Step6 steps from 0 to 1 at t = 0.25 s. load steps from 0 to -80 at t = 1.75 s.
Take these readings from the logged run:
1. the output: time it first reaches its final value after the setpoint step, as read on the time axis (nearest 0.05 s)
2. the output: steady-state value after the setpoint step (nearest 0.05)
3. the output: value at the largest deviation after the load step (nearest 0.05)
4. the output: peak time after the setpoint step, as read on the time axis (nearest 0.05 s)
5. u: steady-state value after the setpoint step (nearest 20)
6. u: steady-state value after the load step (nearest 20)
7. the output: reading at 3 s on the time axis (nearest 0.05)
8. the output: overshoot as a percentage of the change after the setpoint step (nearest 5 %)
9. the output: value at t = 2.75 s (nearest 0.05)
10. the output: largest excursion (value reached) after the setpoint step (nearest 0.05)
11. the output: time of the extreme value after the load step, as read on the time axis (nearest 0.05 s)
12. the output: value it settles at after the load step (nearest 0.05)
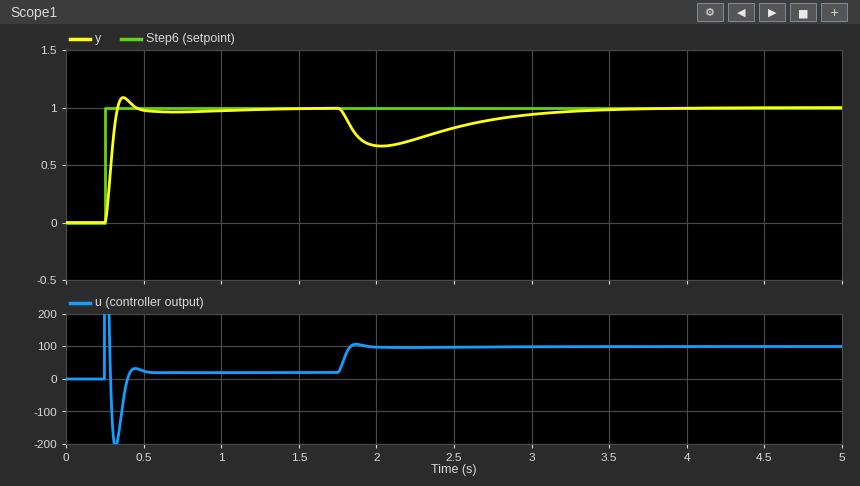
0.35 s
1.00
0.65
0.35 s
20
100
0.95
10 %
0.90
1.10
2.05 s
1.00
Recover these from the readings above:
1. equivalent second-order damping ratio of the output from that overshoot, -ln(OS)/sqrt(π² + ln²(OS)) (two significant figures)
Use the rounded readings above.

0.59
